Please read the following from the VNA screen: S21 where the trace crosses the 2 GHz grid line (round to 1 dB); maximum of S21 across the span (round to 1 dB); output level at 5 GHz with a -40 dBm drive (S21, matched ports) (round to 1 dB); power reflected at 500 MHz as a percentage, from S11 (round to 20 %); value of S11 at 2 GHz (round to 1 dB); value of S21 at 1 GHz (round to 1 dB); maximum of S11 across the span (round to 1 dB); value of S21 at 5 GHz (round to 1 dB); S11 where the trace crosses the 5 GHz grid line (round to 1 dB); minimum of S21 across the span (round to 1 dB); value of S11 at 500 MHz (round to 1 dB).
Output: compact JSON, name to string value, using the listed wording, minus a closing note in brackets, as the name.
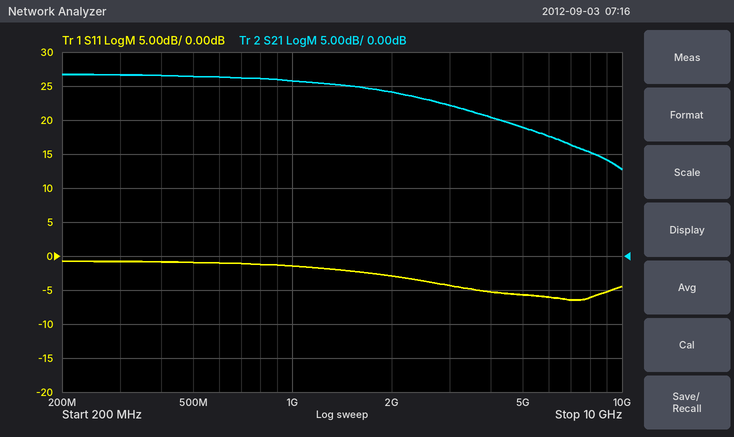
{"S21 where the trace crosses the 2 GHz grid line": "24 dB", "maximum of S21 across the span": "27 dB", "output level at 5 GHz with a -40 dBm drive (S21, matched ports)": "-21 dBm", "power reflected at 500 MHz as a percentage, from S11": "80 %", "value of S11 at 2 GHz": "-3 dB", "value of S21 at 1 GHz": "26 dB", "maximum of S11 across the span": "-1 dB", "value of S21 at 5 GHz": "19 dB", "S11 where the trace crosses the 5 GHz grid line": "-6 dB", "minimum of S21 across the span": "13 dB", "value of S11 at 500 MHz": "-1 dB"}
